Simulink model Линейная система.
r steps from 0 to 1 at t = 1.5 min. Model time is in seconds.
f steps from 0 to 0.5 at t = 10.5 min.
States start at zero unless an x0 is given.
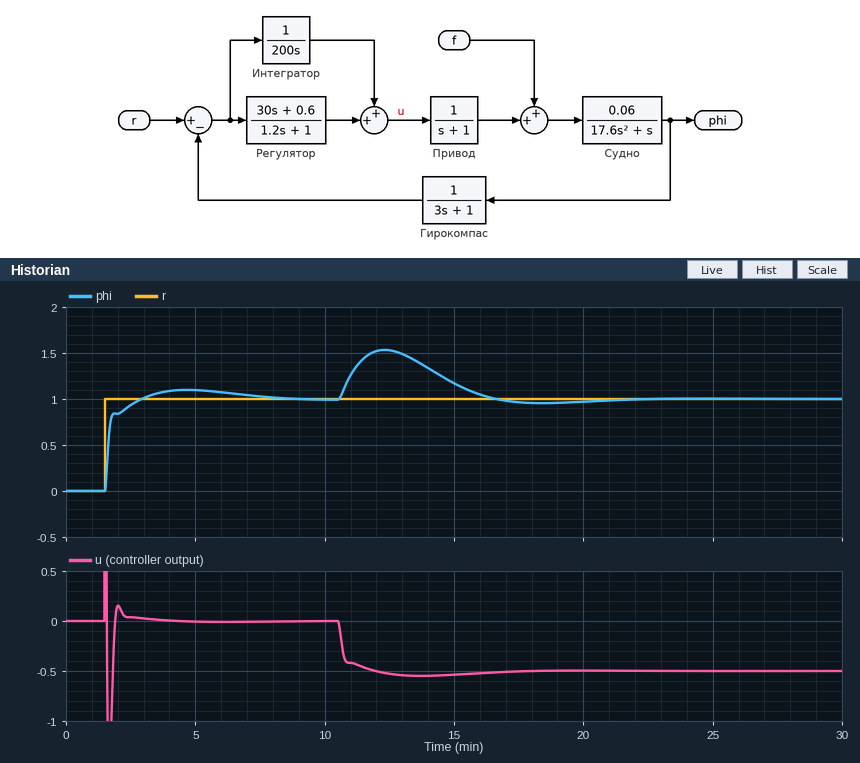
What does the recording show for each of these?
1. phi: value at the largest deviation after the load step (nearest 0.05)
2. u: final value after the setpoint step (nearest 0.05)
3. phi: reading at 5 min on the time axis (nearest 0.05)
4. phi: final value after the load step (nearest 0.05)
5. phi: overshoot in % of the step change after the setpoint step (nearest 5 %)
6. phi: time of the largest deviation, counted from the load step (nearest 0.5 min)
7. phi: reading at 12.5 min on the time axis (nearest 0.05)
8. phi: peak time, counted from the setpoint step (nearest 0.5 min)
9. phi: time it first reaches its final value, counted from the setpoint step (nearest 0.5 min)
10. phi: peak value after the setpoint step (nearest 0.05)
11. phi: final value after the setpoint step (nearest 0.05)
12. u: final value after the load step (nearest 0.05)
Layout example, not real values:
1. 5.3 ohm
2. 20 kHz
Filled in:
1. 1.55
2. 0.00
3. 1.10
4. 1.00
5. 10 %
6. 2.0 min
7. 1.55
8. 3.0 min
9. 1.5 min
10. 1.10
11. 1.00
12. -0.50
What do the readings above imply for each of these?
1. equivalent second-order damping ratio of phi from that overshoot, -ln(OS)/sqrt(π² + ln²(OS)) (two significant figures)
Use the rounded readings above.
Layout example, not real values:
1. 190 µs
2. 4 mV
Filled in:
1. 0.59
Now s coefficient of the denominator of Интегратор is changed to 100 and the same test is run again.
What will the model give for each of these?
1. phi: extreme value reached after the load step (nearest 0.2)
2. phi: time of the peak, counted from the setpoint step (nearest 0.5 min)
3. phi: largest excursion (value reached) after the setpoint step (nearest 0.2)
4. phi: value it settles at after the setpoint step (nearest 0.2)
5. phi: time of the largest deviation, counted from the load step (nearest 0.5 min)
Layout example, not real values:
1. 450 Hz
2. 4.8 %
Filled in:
1. 1.4
2. 2.5 min
3. 1.2
4. 1.0
5. 1.5 min
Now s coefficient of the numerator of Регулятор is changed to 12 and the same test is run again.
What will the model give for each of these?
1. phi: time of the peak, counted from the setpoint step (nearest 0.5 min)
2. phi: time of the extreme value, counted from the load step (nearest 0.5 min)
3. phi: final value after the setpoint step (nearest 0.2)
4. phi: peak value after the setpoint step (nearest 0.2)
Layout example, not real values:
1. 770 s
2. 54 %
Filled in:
1. 2.0 min
2. 1.5 min
3. 1.0
4. 1.2
